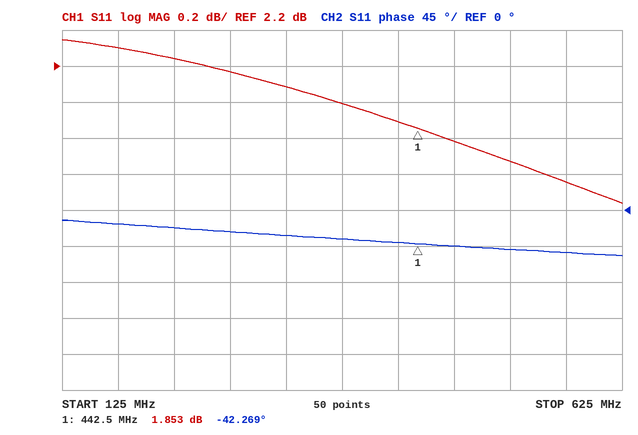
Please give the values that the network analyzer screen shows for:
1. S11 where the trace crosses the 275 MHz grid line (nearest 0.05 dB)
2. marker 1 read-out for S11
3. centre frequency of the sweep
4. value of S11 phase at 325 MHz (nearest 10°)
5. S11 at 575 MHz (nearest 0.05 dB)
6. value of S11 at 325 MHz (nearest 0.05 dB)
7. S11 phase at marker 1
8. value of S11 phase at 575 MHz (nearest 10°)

2.15 dB
1.853 dB
375 MHz
-30°
1.55 dB
2.10 dB
-42.269°
-50°
